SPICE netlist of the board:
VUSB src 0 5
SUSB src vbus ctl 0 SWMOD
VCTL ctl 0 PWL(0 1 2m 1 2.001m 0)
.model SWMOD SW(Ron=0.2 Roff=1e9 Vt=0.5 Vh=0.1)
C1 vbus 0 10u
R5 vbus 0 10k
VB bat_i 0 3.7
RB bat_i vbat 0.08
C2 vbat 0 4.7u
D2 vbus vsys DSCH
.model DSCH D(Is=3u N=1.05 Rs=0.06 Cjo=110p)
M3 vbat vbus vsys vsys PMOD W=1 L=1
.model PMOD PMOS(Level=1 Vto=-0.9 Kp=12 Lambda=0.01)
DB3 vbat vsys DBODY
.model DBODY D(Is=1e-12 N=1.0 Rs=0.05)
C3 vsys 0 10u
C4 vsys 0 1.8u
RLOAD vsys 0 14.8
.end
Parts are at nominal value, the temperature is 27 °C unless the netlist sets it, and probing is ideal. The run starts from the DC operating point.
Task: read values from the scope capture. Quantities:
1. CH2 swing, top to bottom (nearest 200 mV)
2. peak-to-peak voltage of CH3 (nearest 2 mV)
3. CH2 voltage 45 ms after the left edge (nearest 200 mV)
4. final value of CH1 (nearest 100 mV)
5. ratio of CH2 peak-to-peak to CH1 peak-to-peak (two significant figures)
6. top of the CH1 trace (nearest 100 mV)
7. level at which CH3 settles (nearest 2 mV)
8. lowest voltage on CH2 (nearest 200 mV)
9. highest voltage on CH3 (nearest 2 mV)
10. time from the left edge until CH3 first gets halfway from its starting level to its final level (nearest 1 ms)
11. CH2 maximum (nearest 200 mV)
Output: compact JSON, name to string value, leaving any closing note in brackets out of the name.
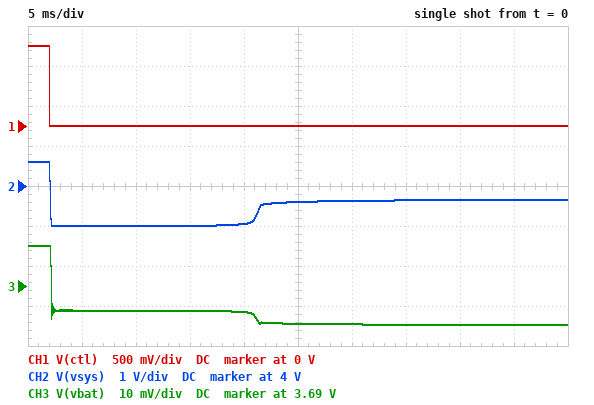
{"CH2 swing, top to bottom": "1.6 V", "peak-to-peak voltage of CH3": "20 mV", "CH2 voltage 45 ms after the left edge": "3.6 V", "final value of CH1": "0 V", "ratio of CH2 peak-to-peak to CH1 peak-to-peak": "1.6", "top of the CH1 trace": "1.0 V", "level at which CH3 settles": "3.680 V", "lowest voltage on CH2": "3.0 V", "highest voltage on CH3": "3.700 V", "time from the left edge until CH3 first gets halfway from its starting level to its final level": "2 ms", "CH2 maximum": "4.6 V"}
